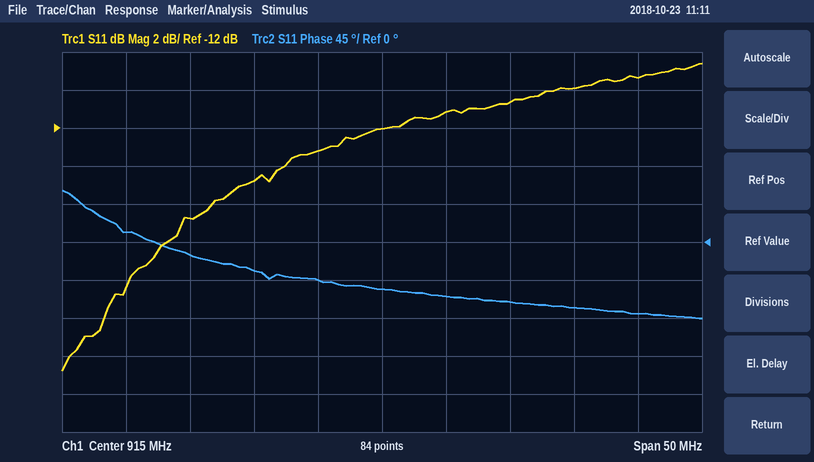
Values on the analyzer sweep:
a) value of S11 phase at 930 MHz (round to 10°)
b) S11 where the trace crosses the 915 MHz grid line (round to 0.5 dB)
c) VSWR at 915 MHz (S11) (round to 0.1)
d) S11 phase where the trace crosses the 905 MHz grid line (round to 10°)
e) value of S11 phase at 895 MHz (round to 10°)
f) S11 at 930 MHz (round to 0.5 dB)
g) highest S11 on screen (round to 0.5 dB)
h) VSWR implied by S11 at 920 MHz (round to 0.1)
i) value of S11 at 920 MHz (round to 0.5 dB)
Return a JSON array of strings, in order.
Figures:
["-80°", "-12.0 dB", "1.7", "-30°", "10°", "-10.0 dB", "-8.5 dB", "1.8", "-11.0 dB"]
